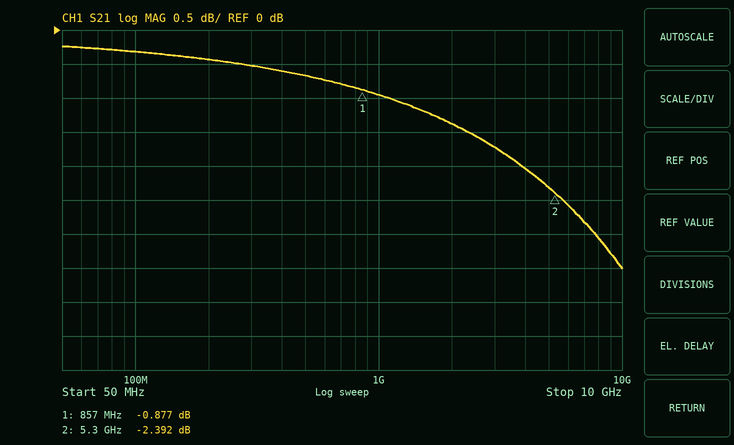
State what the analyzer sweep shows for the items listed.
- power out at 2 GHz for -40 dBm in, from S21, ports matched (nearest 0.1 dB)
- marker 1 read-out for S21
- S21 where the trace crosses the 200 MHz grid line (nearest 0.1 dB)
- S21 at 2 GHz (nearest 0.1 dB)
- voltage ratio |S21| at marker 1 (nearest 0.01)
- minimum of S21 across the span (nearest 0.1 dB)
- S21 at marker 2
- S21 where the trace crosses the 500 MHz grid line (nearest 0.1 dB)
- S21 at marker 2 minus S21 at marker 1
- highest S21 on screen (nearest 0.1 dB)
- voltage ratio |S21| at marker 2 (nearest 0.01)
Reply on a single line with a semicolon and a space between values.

-41.4 dBm; -0.877 dB; -0.4 dB; -1.4 dB; 0.90; -3.5 dB; -2.392 dB; -0.7 dB; -1.515 dB; -0.2 dB; 0.76
